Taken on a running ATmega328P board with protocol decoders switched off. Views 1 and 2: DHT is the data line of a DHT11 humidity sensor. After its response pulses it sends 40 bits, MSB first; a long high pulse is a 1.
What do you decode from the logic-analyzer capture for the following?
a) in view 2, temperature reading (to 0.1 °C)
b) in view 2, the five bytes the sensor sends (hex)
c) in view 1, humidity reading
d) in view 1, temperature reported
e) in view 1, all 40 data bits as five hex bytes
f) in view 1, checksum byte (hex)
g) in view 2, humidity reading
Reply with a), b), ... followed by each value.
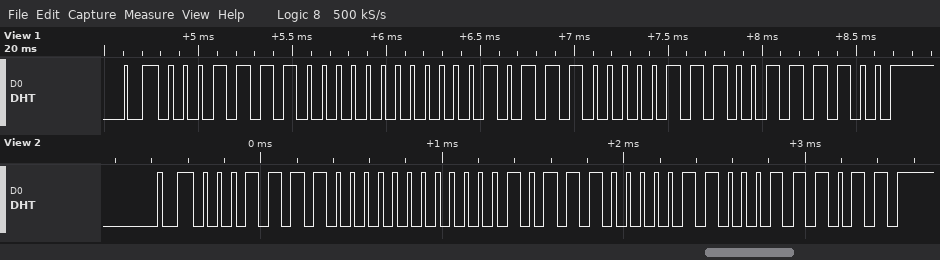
a) 23.6 °C
b) 1E 00 17 06 3B
c) 30 %
d) 23.7 °C
e) 1E 00 17 07 3C
f) 0x3C
g) 30 %
